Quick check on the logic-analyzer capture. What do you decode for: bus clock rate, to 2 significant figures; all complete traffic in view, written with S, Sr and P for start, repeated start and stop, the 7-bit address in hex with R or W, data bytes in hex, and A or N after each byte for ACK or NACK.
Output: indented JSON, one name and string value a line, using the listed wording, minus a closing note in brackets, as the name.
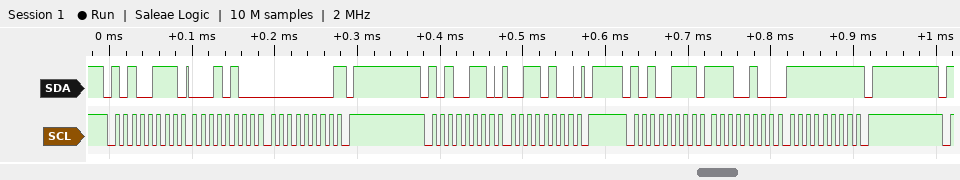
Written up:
{
  "bus clock rate, to 2 significant figures": "100 kHz",
  "all complete traffic in view, written with S, Sr and P for start, repeated start and stop, the 7-bit address in hex with R or W, data bytes in hex, and A or N after each byte for ACK or NACK": "S 53R A 14 A 00 N P S 53W A 34 A P S 53R A E4 A FF N P"
}
